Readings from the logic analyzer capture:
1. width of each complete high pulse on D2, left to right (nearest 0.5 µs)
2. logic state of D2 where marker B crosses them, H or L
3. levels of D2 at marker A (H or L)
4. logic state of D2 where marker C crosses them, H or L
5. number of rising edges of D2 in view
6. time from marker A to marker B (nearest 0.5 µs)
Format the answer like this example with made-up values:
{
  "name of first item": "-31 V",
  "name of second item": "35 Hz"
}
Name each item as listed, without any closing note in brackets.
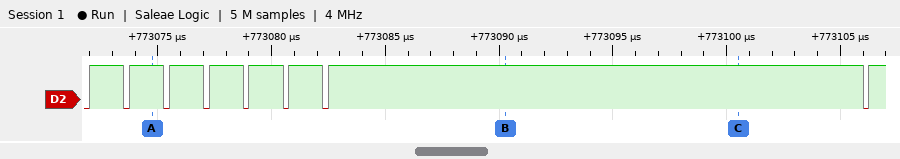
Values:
{
  "width of each complete high pulse on D2, left to right": "1.5 µs, 1.5 µs, 1.5 µs, 1.5 µs, 1.5 µs, 1.5 µs, 23.5 µs",
  "logic state of D2 where marker B crosses them, H or L": "D2=H",
  "levels of D2 at marker A": "D2=H",
  "logic state of D2 where marker C crosses them, H or L": "D2=H",
  "number of rising edges of D2 in view": "8",
  "time from marker A to marker B": "15.5 µs"
}
